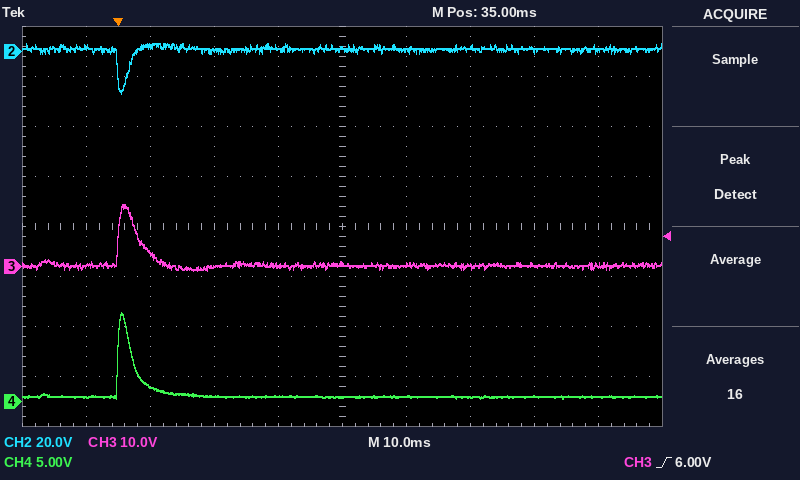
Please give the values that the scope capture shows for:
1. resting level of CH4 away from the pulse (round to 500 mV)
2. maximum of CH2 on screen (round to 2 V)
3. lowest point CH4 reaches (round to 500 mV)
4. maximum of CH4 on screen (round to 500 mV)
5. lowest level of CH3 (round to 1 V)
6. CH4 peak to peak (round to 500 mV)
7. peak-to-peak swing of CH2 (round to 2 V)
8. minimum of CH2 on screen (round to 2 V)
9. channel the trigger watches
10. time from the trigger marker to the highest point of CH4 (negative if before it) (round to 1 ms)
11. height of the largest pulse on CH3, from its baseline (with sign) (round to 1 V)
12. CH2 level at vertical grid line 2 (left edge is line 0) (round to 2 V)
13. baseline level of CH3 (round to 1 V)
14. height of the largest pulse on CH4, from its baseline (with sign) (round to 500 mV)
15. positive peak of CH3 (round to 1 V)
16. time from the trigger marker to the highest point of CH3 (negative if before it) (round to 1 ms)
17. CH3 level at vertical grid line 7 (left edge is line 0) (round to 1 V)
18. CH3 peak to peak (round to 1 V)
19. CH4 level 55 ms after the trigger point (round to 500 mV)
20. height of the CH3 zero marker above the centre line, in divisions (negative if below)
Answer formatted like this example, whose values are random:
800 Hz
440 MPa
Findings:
500 mV
4 V
500 mV
9.0 V
-1 V
8.5 V
20 V
-16 V
CH3
+1 ms
+12 V
2 V
0 V
+8.5 V
12 V
+1 ms
0 V
13 V
500 mV
-0.8 div
